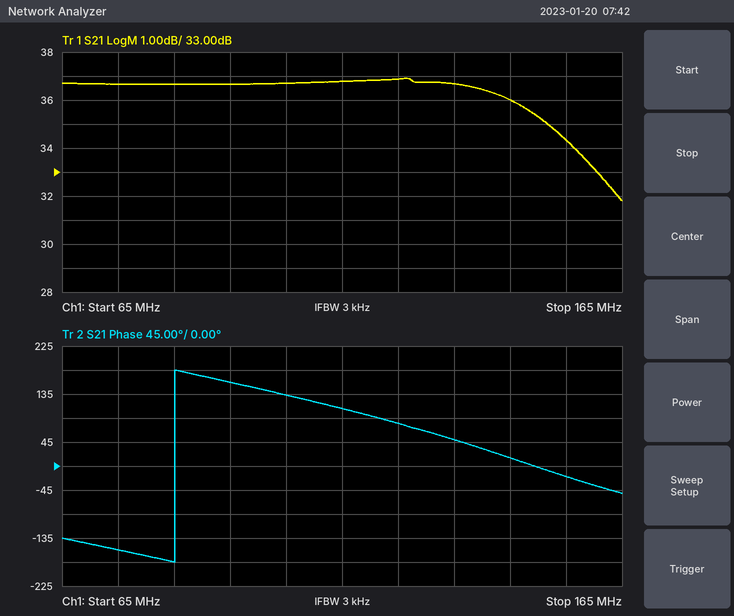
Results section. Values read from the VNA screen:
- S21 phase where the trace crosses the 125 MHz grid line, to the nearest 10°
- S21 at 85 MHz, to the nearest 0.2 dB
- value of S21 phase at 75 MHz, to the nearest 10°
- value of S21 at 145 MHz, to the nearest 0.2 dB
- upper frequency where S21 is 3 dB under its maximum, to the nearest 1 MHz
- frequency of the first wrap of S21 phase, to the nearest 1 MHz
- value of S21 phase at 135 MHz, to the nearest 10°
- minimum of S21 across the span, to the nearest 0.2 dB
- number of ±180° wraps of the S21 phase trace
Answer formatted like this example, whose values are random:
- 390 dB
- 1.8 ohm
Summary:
- 80°
- 36.6 dB
- -160°
- 36.0 dB
- 157 MHz
- 85 MHz
- 50°
- 31.8 dB
- 1
